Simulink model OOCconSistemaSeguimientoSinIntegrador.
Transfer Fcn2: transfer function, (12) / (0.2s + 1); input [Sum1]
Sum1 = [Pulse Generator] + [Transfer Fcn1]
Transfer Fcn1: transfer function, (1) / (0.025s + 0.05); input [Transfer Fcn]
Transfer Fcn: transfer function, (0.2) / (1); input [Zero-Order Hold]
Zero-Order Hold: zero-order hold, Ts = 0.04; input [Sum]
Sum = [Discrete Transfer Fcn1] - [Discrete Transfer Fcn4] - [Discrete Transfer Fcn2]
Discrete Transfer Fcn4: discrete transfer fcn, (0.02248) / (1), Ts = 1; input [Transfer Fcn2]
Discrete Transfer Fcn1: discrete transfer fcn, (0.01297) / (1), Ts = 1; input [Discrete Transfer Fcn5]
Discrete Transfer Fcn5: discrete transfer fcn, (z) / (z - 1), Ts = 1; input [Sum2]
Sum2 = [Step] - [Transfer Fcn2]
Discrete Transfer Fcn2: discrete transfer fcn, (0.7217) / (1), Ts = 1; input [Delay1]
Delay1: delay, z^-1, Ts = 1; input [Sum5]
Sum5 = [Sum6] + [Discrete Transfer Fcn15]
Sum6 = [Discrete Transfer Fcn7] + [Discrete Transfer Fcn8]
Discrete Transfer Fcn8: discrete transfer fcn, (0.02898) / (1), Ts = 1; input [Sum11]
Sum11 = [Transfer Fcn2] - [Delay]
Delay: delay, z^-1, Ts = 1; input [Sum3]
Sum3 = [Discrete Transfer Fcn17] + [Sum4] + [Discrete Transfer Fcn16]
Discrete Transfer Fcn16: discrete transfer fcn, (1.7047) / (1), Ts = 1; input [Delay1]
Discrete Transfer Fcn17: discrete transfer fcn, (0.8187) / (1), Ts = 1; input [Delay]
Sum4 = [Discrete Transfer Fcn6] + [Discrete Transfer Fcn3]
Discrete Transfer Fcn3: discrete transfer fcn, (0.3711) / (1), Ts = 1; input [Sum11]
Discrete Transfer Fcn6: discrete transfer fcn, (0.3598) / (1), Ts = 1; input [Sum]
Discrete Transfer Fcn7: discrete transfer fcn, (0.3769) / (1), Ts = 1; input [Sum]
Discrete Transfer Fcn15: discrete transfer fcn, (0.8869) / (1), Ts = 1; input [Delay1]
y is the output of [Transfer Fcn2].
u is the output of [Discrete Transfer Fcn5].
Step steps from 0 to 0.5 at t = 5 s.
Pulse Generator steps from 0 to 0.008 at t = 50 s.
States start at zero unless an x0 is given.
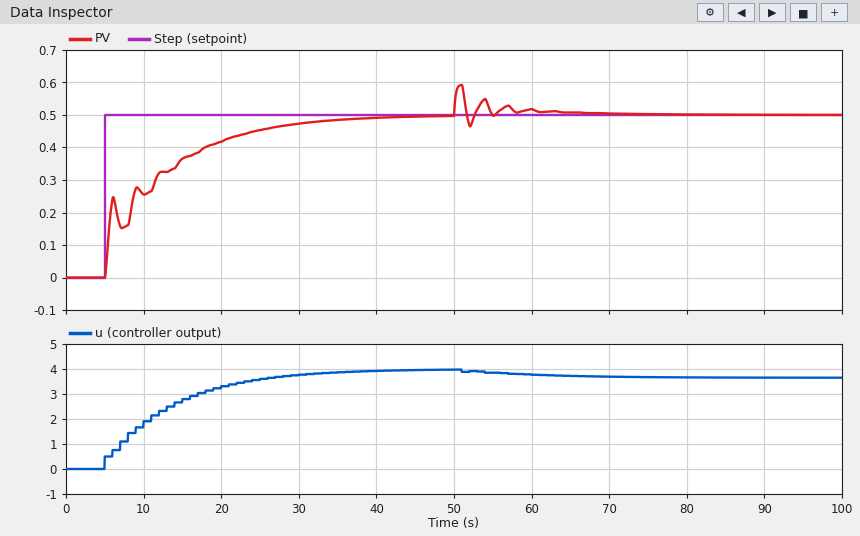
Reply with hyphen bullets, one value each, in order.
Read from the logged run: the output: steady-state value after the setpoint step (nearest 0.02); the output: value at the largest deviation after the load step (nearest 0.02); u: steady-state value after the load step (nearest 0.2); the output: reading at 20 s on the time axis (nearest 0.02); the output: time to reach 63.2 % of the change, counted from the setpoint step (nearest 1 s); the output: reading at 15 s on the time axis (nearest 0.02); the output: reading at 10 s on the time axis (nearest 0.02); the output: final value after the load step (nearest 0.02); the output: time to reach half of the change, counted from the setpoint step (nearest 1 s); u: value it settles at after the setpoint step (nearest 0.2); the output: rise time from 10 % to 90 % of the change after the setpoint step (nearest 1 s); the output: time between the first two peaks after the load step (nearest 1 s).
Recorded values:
- 0.50
- 0.60
- 3.6
- 0.42
- 7 s
- 0.36
- 0.26
- 0.50
- 4 s
- 4.0
- 19 s
- 3 s
